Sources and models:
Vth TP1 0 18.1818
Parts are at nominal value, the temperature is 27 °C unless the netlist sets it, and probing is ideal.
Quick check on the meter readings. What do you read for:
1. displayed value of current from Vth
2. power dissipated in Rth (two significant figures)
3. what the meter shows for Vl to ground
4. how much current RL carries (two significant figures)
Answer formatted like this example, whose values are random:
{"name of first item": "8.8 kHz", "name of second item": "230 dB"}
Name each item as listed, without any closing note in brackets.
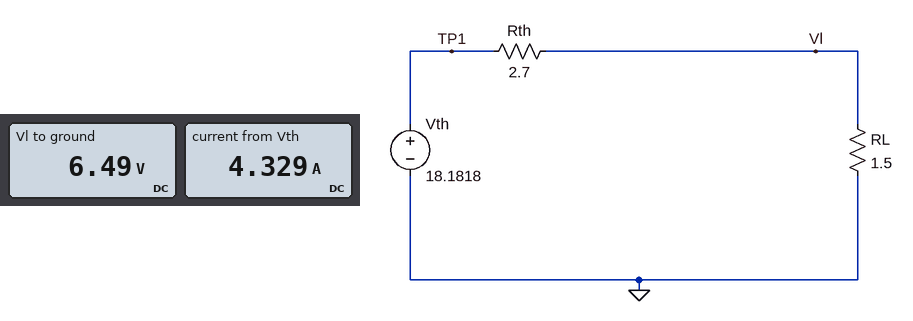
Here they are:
{"displayed value of current from Vth": "4.329 A", "power dissipated in Rth": "51 W", "what the meter shows for Vl to ground": "6.49 V", "how much current RL carries": "4.3 A"}
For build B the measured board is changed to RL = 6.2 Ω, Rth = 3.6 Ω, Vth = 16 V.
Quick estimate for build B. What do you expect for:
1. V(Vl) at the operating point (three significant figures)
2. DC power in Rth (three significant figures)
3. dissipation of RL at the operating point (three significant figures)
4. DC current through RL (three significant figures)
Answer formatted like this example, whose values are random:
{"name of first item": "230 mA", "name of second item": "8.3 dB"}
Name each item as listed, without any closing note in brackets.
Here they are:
{"V(Vl) at the operating point": "10.1 V", "DC power in Rth": "9.60 W", "dissipation of RL at the operating point": "16.5 W", "DC current through RL": "1.63 A"}
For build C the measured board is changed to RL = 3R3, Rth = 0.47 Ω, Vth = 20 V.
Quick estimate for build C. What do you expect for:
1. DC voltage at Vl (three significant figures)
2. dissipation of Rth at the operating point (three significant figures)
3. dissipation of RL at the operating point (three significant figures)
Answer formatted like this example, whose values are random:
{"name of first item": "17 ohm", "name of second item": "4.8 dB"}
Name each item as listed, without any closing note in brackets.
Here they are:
{"DC voltage at Vl": "17.5 V", "dissipation of Rth at the operating point": "13.2 W", "dissipation of RL at the operating point": "92.9 W"}
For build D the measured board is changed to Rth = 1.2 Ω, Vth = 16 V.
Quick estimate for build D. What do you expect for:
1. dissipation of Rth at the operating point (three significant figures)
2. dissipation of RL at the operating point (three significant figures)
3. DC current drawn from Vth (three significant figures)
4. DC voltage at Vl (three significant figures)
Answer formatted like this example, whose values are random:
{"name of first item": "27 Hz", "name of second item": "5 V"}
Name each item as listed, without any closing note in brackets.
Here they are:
{"dissipation of Rth at the operating point": "42.1 W", "dissipation of RL at the operating point": "52.7 W", "DC current drawn from Vth": "5.93 A", "DC voltage at Vl": "8.89 V"}
